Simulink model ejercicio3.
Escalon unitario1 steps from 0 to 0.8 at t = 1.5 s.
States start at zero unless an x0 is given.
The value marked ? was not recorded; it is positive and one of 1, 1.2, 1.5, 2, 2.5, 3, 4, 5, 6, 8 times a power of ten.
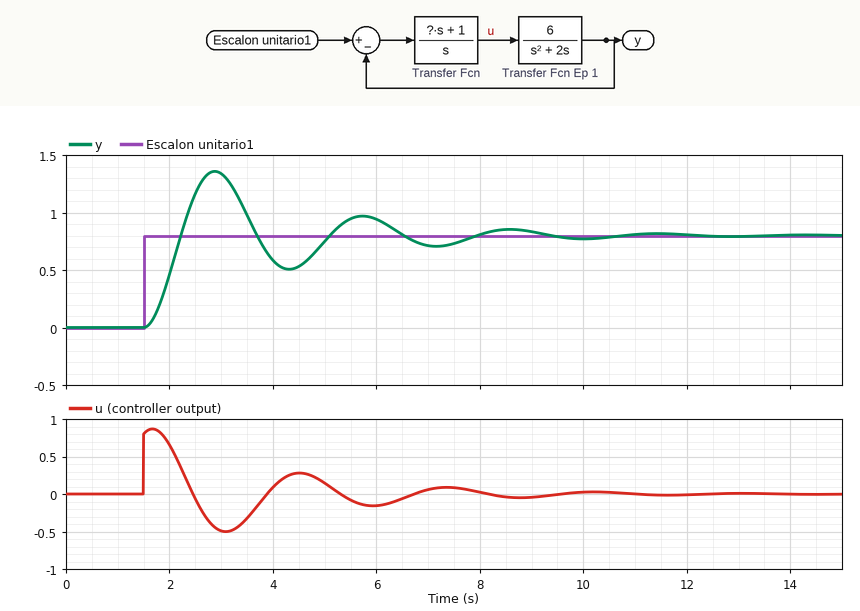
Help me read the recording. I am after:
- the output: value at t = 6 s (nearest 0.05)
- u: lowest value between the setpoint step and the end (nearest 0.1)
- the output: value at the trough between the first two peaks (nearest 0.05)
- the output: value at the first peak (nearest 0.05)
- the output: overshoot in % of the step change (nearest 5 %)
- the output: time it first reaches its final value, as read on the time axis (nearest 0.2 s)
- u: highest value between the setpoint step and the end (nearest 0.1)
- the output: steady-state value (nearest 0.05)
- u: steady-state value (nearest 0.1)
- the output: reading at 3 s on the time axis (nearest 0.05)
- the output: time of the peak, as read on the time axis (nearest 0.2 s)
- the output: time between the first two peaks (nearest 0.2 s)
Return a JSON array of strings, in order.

["0.95", "-0.5", "0.50", "1.35", "70 %", "2.2 s", "0.9", "0.80", "0.0", "1.35", "2.8 s", "2.8 s"]
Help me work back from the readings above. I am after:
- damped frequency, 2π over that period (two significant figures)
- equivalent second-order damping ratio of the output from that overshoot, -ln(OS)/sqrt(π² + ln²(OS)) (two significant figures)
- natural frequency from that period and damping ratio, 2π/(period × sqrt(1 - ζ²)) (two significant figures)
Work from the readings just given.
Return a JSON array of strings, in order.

["2.2 rad/s", "0.11", "2.3 rad/s"]
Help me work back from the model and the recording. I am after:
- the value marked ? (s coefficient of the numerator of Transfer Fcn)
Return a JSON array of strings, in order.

["1"]
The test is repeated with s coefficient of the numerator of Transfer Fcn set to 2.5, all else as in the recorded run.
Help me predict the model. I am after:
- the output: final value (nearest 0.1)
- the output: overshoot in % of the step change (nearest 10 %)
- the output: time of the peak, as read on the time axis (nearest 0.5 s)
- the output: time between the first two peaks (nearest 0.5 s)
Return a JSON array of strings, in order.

["0.8", "60 %", "2.5 s", "1.5 s"]
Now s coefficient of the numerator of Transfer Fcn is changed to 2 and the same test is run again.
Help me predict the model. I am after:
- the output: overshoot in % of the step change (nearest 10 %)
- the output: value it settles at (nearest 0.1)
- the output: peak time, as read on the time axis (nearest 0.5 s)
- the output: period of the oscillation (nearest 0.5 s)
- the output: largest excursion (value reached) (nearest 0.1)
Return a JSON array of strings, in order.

["60 %", "0.8", "2.5 s", "2.0 s", "1.3"]
